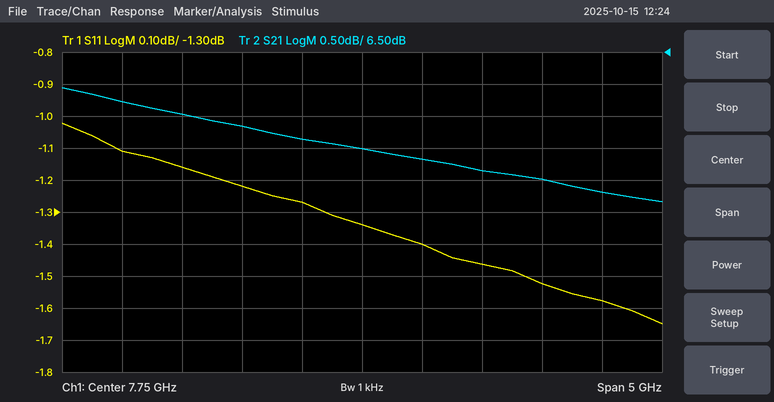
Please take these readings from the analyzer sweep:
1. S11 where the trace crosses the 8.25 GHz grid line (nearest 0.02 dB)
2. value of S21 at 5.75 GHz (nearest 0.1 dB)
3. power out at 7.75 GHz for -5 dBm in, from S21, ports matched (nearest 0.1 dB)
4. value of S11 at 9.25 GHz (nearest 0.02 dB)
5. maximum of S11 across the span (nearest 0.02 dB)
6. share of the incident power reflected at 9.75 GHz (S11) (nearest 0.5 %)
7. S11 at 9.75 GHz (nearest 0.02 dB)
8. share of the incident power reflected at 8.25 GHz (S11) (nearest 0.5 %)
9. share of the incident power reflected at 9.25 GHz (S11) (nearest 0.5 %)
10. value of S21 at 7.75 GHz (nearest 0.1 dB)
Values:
-1.40 dB
5.7 dB
0.0 dBm
-1.52 dB
-1.02 dB
69.5 %
-1.58 dB
72.5 %
70.5 %
5.0 dB
